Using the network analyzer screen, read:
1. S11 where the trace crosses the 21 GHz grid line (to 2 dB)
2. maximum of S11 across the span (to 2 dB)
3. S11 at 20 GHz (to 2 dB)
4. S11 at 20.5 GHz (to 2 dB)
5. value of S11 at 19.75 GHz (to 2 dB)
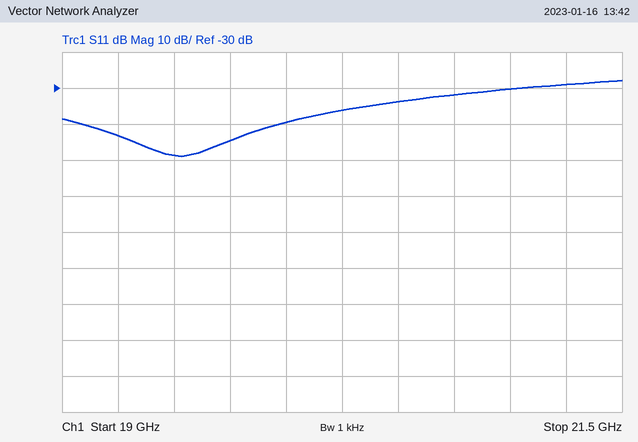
-30 dB
-28 dB
-40 dB
-34 dB
-44 dB
